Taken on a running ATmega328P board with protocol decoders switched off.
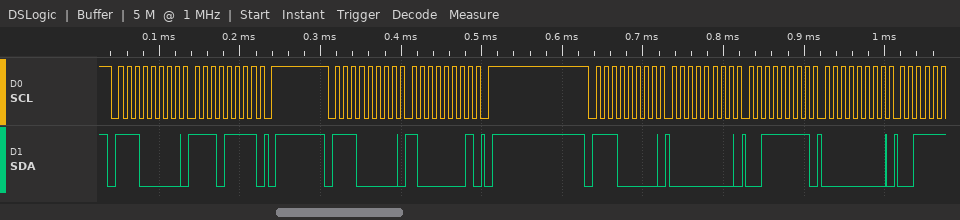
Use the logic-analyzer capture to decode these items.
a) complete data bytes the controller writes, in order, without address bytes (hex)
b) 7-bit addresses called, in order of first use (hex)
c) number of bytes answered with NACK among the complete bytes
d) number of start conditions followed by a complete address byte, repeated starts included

EF 81 00 3F 00
0x70
0
3
